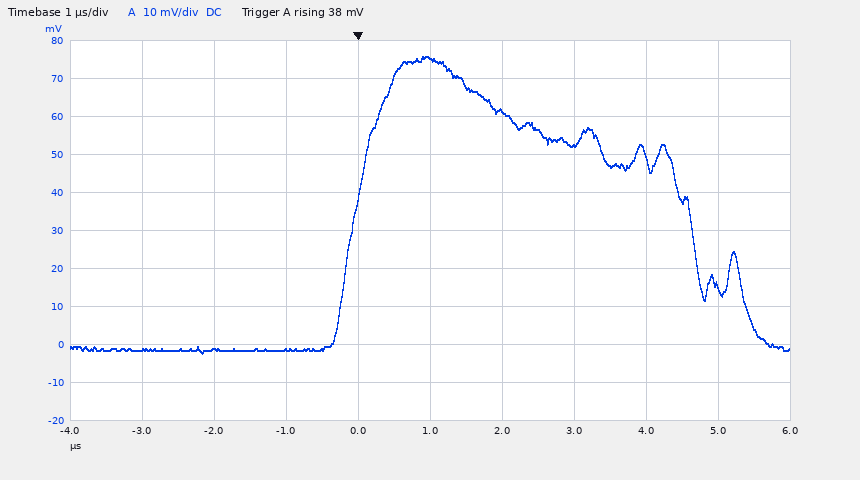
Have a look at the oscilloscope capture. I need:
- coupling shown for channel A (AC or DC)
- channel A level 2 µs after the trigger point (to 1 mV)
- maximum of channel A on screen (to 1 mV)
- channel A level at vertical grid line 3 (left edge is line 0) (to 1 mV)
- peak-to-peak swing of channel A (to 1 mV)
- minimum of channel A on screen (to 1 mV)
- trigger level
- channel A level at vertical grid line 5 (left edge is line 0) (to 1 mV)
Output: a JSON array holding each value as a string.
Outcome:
["DC", "61 mV", "76 mV", "-1 mV", "78 mV", "-2 mV", "38 mV", "75 mV"]
